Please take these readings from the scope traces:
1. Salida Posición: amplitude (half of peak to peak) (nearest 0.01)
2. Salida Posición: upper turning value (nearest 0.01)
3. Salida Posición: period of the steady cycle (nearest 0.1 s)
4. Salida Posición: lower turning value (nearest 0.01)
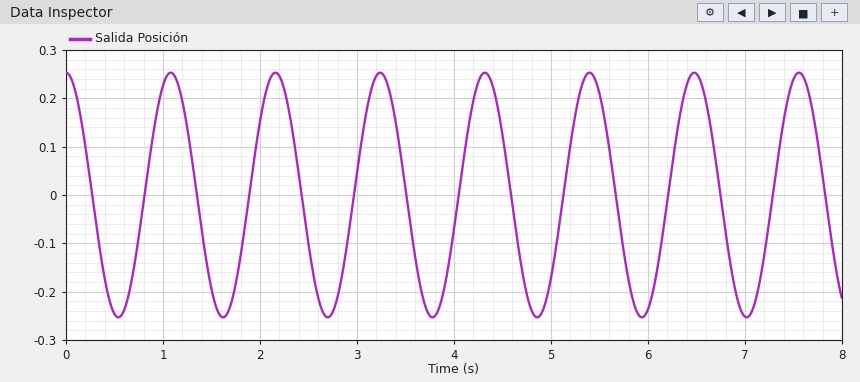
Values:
0.25
0.25
1.1 s
-0.25
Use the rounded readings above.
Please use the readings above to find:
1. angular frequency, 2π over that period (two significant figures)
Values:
5.7 rad/s
